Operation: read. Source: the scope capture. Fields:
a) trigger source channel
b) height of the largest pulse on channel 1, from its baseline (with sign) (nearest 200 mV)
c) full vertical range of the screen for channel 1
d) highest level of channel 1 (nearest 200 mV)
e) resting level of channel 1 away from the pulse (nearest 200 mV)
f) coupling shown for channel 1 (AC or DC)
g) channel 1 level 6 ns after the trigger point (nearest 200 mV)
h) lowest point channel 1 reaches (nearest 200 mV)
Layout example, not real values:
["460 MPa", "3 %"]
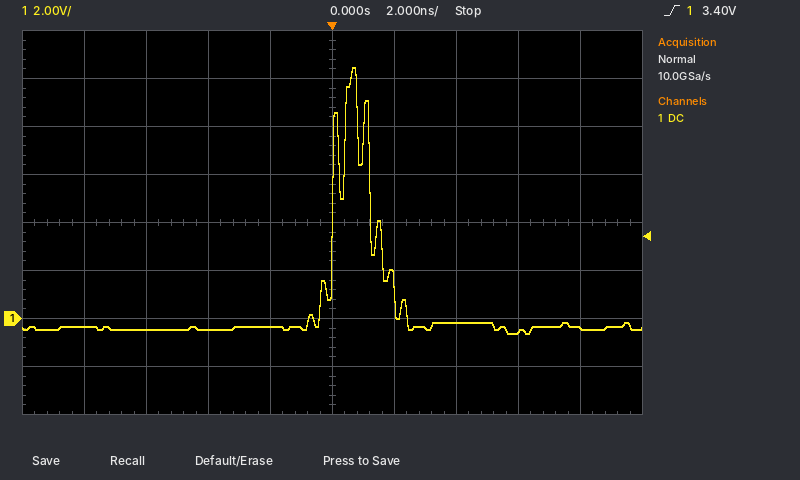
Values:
["channel 1", "+10.8 V", "16 V", "10.4 V", "-400 mV", "DC", "-600 mV", "-600 mV"]
